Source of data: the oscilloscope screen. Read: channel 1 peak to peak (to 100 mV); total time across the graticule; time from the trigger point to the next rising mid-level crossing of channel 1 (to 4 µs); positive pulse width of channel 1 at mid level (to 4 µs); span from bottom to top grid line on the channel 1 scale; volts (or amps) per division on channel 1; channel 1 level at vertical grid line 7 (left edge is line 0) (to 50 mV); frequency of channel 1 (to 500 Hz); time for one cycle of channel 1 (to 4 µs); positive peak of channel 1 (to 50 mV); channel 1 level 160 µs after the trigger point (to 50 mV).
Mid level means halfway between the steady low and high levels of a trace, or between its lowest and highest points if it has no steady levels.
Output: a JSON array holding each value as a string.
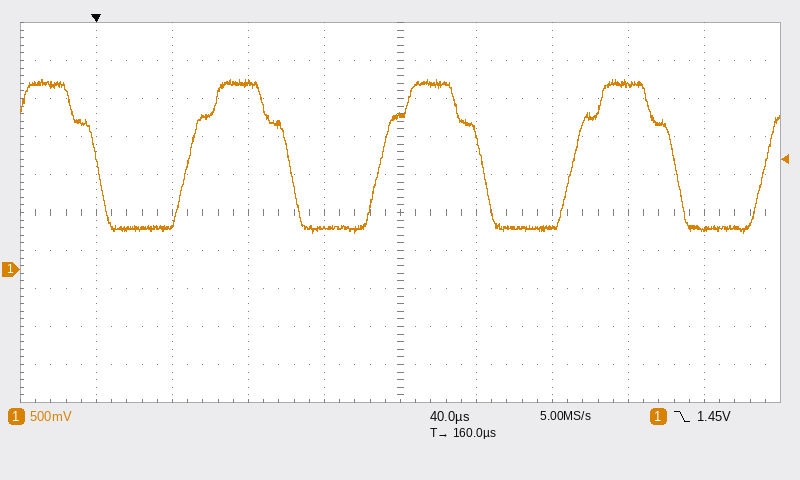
["2.00 V", "400 µs", "48 µs", "52 µs", "5 V", "500 mV", "550 mV", "10.0 kHz", "100 µs", "2.50 V", "2.00 V"]
